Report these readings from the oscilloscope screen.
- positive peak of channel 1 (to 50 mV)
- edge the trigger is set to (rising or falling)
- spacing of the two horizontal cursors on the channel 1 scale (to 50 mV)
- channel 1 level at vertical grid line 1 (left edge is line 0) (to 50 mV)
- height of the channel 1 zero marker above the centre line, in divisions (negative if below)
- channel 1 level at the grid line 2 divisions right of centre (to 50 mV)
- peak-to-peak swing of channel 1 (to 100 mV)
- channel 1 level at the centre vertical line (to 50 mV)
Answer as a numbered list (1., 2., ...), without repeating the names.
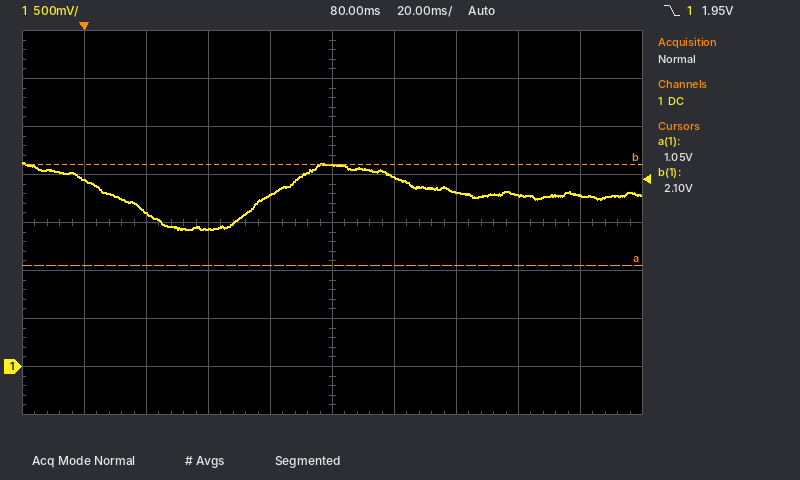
1. 2.10 V
2. falling
3. 1.05 V
4. 1.95 V
5. -3.0 div
6. 1.80 V
7. 700 mV
8. 2.10 V
